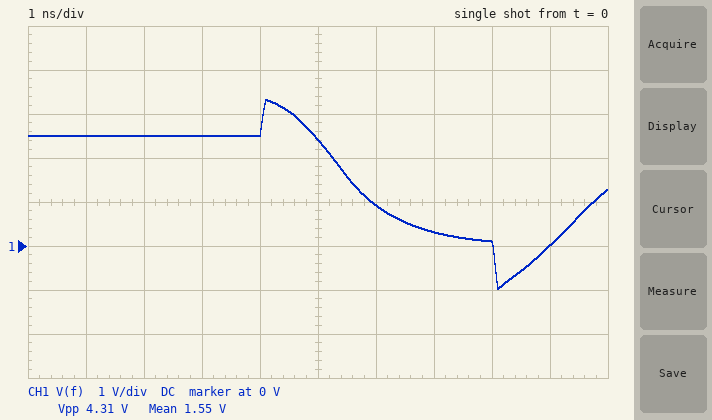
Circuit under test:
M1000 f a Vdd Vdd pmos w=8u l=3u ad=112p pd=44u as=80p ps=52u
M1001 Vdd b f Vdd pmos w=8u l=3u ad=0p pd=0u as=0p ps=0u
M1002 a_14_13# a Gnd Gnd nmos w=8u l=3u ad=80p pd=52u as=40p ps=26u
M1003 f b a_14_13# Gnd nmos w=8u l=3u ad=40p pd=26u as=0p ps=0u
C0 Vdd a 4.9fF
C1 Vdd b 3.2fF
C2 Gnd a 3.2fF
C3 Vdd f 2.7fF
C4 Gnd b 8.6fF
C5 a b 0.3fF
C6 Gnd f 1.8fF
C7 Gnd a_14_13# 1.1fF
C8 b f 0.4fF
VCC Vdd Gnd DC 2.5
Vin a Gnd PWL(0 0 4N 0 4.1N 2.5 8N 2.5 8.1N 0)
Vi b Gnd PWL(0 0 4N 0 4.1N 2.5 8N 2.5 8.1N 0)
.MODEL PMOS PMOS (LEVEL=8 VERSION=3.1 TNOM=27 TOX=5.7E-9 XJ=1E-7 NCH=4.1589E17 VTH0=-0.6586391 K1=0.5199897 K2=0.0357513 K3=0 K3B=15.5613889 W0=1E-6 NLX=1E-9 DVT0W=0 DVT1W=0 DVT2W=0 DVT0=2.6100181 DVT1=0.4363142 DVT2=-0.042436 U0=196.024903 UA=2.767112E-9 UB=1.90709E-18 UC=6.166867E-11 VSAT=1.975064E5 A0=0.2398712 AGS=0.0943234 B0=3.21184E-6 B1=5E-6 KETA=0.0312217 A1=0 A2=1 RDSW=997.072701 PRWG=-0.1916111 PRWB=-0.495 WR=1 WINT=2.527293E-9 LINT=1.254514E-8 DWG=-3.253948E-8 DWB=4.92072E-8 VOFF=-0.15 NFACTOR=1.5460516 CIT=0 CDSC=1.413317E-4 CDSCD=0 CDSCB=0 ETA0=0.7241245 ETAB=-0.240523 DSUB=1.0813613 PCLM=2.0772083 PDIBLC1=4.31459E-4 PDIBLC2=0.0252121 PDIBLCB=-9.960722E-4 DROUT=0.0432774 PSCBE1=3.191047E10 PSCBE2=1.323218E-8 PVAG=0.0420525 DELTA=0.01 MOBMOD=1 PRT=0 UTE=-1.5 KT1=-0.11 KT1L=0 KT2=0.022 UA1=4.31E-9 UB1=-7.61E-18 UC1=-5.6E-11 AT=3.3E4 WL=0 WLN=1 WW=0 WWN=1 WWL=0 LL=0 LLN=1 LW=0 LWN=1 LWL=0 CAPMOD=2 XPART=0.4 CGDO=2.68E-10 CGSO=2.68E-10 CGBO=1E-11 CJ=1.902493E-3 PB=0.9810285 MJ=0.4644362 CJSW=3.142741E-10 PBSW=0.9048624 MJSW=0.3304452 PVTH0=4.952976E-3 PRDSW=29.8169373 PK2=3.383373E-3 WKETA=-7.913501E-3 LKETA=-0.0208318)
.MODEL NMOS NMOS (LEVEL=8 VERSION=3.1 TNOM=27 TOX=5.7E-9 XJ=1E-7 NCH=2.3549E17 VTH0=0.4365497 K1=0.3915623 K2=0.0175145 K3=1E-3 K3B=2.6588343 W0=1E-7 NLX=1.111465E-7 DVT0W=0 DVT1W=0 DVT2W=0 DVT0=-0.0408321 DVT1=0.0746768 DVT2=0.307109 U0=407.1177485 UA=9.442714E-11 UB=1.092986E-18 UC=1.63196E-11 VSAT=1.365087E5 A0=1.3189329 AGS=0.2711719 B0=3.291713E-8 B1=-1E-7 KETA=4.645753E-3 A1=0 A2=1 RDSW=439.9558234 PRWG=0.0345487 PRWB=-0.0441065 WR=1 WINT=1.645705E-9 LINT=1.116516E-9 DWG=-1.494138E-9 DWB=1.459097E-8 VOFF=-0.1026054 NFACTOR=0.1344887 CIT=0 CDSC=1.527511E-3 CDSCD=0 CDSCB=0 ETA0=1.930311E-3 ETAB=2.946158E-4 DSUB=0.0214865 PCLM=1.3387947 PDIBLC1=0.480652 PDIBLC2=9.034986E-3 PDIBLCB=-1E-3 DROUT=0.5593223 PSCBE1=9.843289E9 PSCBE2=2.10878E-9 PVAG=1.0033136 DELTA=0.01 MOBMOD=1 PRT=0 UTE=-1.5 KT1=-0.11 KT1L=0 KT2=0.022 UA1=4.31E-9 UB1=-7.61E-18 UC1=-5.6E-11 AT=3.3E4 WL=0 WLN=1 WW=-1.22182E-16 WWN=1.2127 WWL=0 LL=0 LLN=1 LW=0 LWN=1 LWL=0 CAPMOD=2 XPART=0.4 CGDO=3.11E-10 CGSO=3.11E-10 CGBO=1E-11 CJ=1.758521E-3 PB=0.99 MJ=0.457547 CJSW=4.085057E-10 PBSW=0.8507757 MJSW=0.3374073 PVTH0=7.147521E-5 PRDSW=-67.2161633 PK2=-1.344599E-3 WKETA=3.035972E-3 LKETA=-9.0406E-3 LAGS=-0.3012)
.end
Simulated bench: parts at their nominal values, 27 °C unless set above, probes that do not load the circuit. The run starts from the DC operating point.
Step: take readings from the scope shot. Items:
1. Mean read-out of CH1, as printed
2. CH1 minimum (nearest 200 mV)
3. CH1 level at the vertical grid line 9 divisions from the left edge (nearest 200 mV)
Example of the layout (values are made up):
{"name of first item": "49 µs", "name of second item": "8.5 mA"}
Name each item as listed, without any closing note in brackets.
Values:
{"Mean read-out of CH1, as printed": "1.55 V", "CH1 minimum": "-1.0 V", "CH1 level at the vertical grid line 9 divisions from the left edge": "0 V"}
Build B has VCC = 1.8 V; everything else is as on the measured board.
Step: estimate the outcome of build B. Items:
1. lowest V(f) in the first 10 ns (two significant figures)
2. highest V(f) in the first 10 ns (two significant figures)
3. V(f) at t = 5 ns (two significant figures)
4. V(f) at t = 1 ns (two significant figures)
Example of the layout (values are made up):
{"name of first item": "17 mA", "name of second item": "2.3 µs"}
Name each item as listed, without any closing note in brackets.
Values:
{"lowest V(f) in the first 10 ns": "-850 mV", "highest V(f) in the first 10 ns": "2.5 V", "V(f) at t = 5 ns": "1.4 V", "V(f) at t = 1 ns": "1.8 V"}
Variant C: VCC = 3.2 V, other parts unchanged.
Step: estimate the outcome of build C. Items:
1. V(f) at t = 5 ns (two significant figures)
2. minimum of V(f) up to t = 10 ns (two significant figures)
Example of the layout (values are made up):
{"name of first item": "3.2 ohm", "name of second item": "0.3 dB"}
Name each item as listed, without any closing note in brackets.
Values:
{"V(f) at t = 5 ns": "3.2 V", "minimum of V(f) up to t = 10 ns": "-1.1 V"}
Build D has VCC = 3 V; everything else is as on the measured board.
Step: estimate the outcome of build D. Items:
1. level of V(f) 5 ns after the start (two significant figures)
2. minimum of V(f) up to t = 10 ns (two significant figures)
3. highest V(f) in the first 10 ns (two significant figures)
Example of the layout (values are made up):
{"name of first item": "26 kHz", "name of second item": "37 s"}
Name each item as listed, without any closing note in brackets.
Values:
{"level of V(f) 5 ns after the start": "3.0 V", "minimum of V(f) up to t = 10 ns": "-1.1 V", "highest V(f) in the first 10 ns": "3.8 V"}
